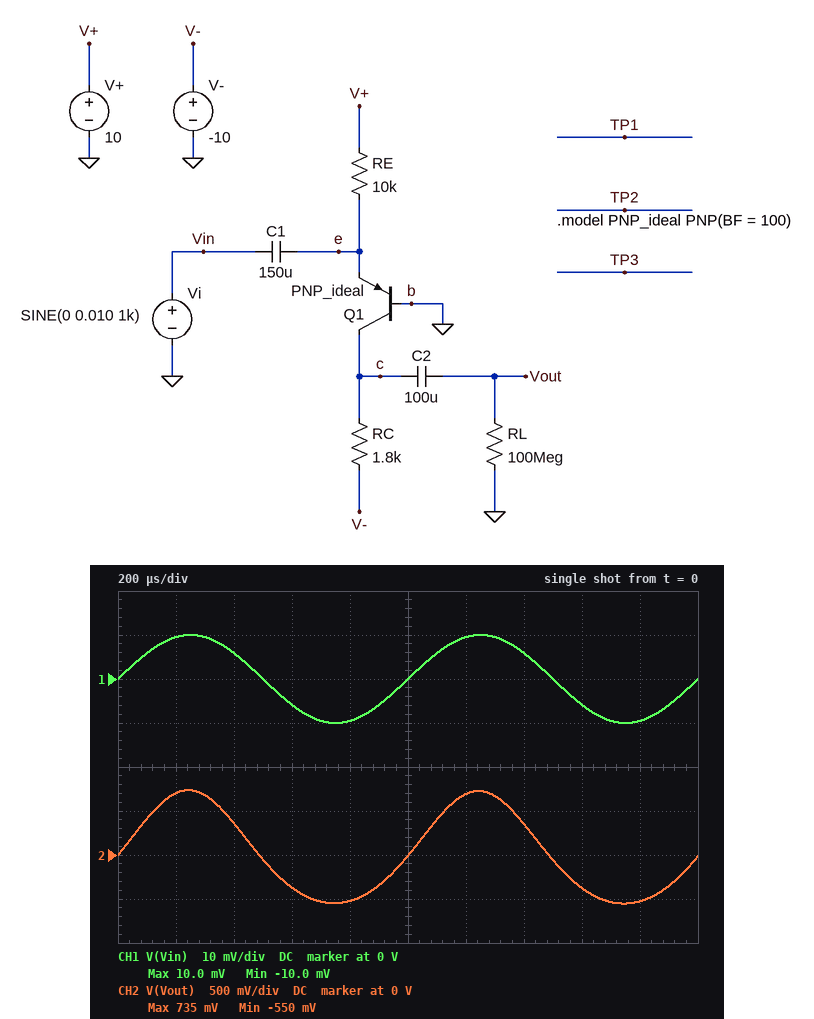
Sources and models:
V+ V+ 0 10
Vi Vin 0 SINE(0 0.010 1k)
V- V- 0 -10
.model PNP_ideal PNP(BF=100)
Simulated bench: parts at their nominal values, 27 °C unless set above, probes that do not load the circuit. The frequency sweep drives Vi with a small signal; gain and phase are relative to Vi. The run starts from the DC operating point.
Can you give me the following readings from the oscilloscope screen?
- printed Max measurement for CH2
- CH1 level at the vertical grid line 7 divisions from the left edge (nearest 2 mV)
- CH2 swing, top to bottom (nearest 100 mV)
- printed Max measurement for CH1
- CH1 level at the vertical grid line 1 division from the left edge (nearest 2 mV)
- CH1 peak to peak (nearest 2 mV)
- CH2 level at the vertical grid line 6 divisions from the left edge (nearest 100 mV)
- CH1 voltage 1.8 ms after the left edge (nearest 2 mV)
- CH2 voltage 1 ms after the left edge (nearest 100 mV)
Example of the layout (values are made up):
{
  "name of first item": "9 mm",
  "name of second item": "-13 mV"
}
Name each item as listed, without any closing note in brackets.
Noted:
{
  "printed Max measurement for CH2": "735 mV",
  "CH1 level at the vertical grid line 7 divisions from the left edge": "6 mV",
  "CH2 swing, top to bottom": "1.3 V",
  "printed Max measurement for CH1": "10.0 mV",
  "CH1 level at the vertical grid line 1 division from the left edge": "10 mV",
  "CH1 peak to peak": "20 mV",
  "CH2 level at the vertical grid line 6 divisions from the left edge": "700 mV",
  "CH1 voltage 1.8 ms after the left edge": "-10 mV",
  "CH2 voltage 1 ms after the left edge": "0 V"
}
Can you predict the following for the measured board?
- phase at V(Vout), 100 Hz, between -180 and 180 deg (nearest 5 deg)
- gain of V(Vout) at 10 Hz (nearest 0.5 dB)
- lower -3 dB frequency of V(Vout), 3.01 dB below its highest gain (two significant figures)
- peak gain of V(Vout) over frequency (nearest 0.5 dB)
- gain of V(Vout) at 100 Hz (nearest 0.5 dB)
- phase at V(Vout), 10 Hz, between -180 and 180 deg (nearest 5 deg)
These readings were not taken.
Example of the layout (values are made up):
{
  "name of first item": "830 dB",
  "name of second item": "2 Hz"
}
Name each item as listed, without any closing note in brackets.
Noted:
{
  "phase at V(Vout), 100 Hz, between -180 and 180 deg": "20 deg",
  "gain of V(Vout) at 10 Hz": "24.0 dB",
  "lower -3 dB frequency of V(Vout), 3.01 dB below its highest gain": "38 Hz",
  "peak gain of V(Vout) over frequency": "36.0 dB",
  "gain of V(Vout) at 100 Hz": "35.5 dB",
  "phase at V(Vout), 10 Hz, between -180 and 180 deg": "75 deg"
}
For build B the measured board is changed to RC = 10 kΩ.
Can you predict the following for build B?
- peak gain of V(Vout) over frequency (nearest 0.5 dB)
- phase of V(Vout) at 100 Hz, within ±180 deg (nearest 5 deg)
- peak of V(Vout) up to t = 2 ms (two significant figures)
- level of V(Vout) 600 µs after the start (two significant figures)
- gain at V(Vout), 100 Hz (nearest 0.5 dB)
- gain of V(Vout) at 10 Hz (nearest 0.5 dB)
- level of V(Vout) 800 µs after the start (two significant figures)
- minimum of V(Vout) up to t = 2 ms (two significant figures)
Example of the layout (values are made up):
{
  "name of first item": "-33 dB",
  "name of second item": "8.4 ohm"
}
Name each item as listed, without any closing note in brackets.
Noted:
{
  "peak gain of V(Vout) over frequency": "51.0 dB",
  "phase of V(Vout) at 100 Hz, within ±180 deg": "20 deg",
  "peak of V(Vout) up to t = 2 ms": "1.6 V",
  "level of V(Vout) 600 µs after the start": "-2.0 V",
  "gain at V(Vout), 100 Hz": "50.5 dB",
  "gain of V(Vout) at 10 Hz": "39.0 dB",
  "level of V(Vout) 800 µs after the start": "-2.9 V",
  "minimum of V(Vout) up to t = 2 ms": "-3.0 V"
}
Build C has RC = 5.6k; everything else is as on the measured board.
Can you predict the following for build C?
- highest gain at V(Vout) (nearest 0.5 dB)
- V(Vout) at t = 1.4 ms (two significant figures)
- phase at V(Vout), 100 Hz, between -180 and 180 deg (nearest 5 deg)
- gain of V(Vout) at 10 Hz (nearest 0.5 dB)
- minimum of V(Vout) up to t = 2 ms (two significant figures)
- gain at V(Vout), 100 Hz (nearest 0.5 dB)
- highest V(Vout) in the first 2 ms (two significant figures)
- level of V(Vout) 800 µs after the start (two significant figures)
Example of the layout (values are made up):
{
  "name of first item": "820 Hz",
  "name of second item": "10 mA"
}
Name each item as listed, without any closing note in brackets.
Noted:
{
  "highest gain at V(Vout)": "46.0 dB",
  "V(Vout) at t = 1.4 ms": "1.1 V",
  "phase at V(Vout), 100 Hz, between -180 and 180 deg": "20 deg",
  "gain of V(Vout) at 10 Hz": "34.0 dB",
  "minimum of V(Vout) up to t = 2 ms": "-1.7 V",
  "gain at V(Vout), 100 Hz": "45.5 dB",
  "highest V(Vout) in the first 2 ms": "2.3 V",
  "level of V(Vout) 800 µs after the start": "-1.6 V"
}
